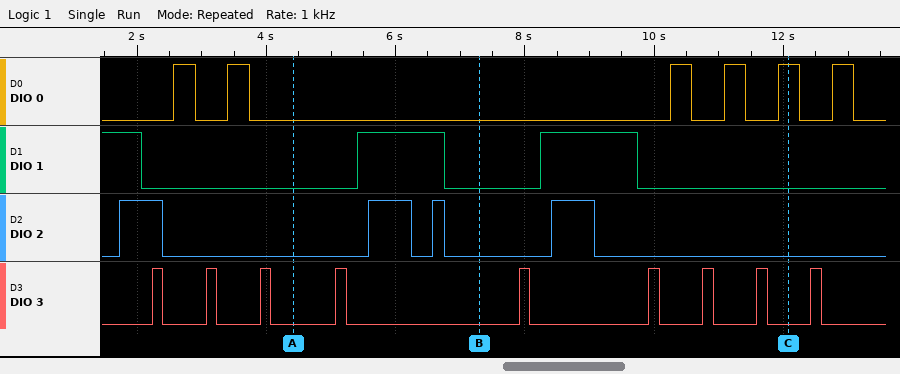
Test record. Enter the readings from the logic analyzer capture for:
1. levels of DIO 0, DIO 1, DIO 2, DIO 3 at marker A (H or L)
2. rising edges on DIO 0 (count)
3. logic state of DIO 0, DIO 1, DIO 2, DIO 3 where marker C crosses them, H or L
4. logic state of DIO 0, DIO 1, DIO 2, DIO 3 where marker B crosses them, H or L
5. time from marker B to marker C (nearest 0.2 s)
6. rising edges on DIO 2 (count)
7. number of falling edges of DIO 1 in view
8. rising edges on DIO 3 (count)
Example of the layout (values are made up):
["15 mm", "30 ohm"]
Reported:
["DIO 0=L, DIO 1=L, DIO 2=L, DIO 3=L", "6", "DIO 0=H, DIO 1=L, DIO 2=L, DIO 3=L", "DIO 0=L, DIO 1=L, DIO 2=L, DIO 3=L", "4.8 s", "4", "3", "9"]
